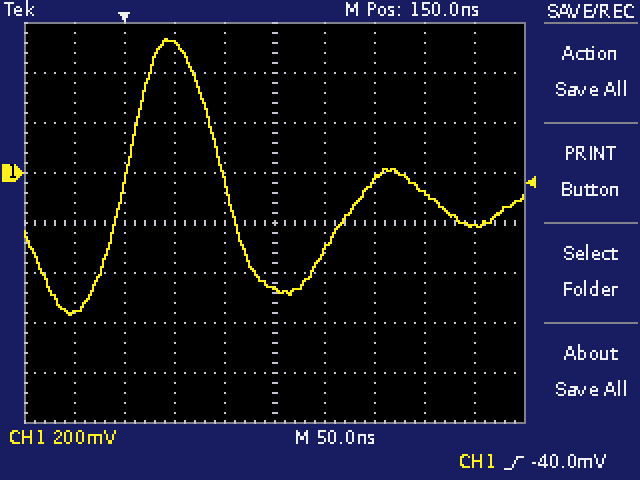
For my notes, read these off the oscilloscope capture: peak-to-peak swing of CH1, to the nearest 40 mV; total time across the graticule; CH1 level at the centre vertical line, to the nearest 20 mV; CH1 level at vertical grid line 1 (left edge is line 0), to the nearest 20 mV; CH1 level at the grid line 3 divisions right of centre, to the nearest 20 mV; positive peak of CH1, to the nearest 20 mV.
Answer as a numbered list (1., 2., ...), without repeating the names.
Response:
1. 1.12 V
2. 500 ns
3. -460 mV
4. -560 mV
5. -80 mV
6. 540 mV
